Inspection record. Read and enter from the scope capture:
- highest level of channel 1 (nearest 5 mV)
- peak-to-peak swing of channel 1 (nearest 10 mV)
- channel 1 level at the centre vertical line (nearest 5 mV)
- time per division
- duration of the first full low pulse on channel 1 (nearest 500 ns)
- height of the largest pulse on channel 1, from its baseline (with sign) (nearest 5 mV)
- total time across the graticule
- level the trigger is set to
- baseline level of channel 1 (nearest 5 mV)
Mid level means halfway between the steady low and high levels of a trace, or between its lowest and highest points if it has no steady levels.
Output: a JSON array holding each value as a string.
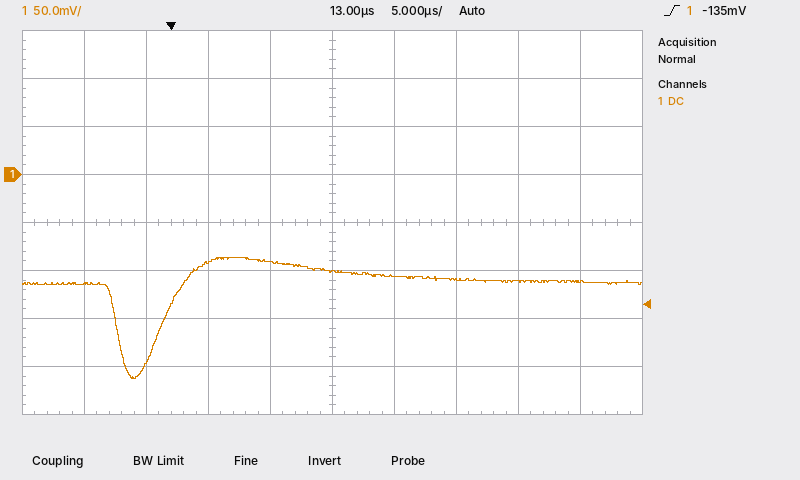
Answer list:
["-85 mV", "130 mV", "-100 mV", "5 µs", "4.0 µs", "-100 mV", "50 µs", "-135 mV", "-110 mV"]
